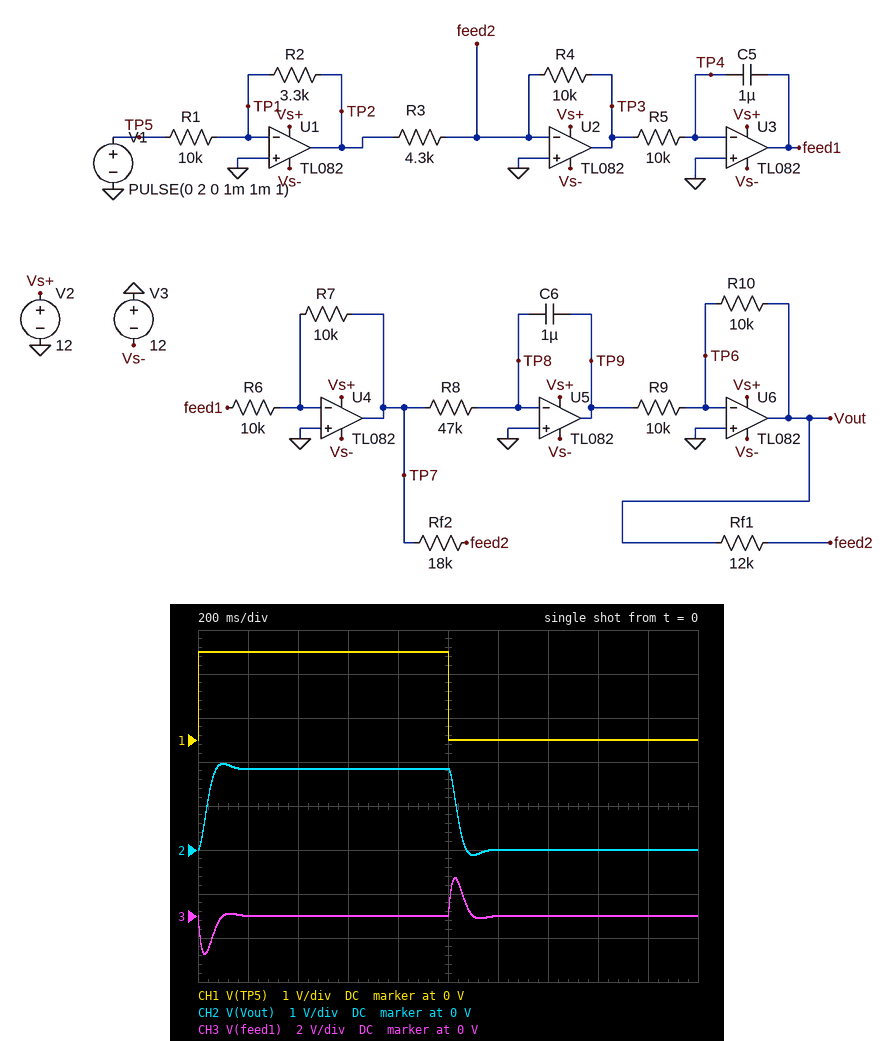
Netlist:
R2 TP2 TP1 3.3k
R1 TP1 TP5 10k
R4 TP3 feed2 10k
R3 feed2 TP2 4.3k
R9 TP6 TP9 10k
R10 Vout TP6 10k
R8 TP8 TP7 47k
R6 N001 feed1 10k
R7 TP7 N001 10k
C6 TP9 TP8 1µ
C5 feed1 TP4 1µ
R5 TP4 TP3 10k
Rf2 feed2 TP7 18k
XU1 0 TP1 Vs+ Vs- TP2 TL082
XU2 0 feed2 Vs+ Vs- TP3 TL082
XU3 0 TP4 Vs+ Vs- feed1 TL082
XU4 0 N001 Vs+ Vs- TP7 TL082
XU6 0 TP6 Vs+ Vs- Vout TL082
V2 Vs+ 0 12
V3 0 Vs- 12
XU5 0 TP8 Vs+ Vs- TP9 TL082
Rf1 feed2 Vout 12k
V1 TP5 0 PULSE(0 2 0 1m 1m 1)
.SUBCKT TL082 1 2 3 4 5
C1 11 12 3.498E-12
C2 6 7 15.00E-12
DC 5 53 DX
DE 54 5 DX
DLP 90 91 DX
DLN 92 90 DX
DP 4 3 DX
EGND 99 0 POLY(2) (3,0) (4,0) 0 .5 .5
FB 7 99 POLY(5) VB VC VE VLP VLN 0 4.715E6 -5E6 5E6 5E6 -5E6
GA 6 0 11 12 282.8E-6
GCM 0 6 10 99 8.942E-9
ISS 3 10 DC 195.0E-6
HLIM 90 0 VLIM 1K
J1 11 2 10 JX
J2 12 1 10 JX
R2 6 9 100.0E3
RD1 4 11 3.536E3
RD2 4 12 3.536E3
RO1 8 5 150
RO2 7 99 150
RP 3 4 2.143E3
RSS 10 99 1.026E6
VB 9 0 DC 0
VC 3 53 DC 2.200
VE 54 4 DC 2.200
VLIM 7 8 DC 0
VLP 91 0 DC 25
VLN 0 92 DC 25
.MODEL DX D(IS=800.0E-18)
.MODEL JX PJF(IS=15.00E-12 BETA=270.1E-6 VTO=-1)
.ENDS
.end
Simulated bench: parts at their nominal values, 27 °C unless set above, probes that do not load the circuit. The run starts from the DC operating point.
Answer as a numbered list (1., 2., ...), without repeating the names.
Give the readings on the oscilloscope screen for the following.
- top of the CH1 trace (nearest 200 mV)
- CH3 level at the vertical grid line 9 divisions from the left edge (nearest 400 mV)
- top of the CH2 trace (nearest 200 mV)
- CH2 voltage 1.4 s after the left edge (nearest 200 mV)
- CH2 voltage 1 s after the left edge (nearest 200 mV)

1. 2.0 V
2. 0 V
3. 2.0 V
4. 0 V
5. 1.8 V
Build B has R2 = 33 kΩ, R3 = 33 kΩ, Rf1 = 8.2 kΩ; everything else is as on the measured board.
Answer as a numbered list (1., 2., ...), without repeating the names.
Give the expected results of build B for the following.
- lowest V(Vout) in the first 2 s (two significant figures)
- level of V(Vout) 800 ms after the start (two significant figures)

1. -210 mV
2. 1.6 V
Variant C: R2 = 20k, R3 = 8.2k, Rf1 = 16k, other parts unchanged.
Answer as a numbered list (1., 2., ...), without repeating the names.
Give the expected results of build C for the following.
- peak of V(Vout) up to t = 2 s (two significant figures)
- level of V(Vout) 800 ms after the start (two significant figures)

1. 8.0 V
2. 7.8 V
